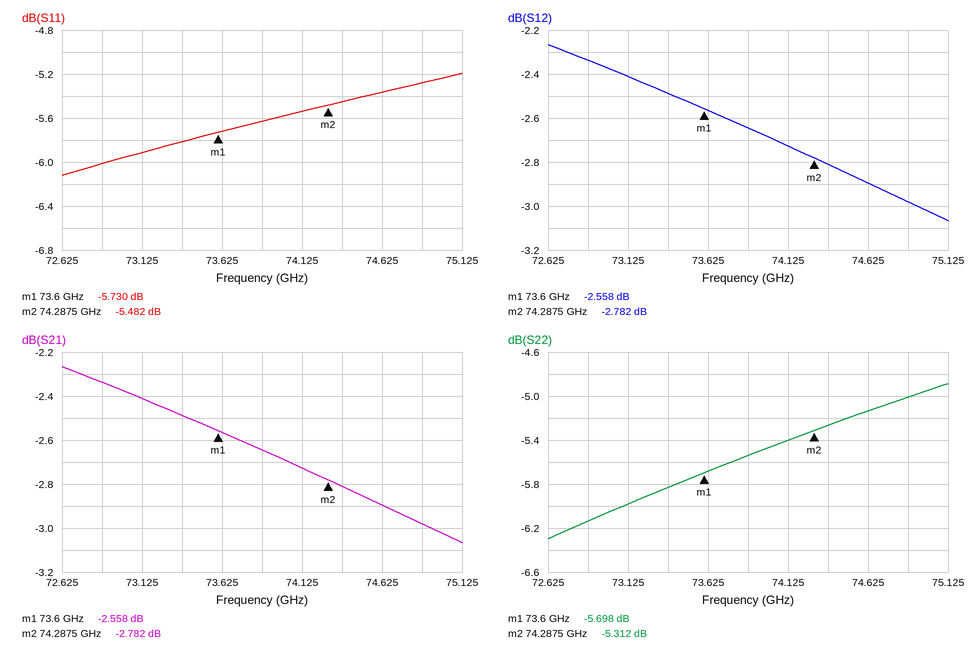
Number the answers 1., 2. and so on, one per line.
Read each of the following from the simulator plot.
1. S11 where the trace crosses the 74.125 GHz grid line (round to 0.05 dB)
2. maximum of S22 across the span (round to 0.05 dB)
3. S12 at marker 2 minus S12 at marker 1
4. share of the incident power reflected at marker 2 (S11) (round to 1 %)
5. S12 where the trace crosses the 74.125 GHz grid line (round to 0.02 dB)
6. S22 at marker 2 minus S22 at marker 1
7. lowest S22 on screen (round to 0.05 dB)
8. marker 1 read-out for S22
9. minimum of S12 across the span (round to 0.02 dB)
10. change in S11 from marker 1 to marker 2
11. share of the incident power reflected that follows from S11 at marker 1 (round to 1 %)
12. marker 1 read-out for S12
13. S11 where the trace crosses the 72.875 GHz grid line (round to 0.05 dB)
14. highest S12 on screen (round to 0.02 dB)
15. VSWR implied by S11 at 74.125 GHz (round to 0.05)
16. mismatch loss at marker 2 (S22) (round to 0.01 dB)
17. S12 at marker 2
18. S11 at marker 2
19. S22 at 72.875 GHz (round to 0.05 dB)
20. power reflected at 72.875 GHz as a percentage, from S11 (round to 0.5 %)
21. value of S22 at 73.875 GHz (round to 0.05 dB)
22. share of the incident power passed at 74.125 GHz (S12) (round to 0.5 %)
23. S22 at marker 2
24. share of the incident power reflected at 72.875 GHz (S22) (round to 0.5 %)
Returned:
1. -5.55 dB
2. -4.90 dB
3. -0.224 dB
4. 28 %
5. -2.72 dB
6. 0.386 dB
7. -6.30 dB
8. -5.698 dB
9. -3.06 dB
10. 0.248 dB
11. 27 %
12. -2.558 dB
13. -6.00 dB
14. -2.26 dB
15. 3.25
16. 1.51 dB
17. -2.782 dB
18. -5.482 dB
19. -6.15 dB
20. 25.0 %
21. -5.55 dB
22. 53.5 %
23. -5.312 dB
24. 24.5 %
